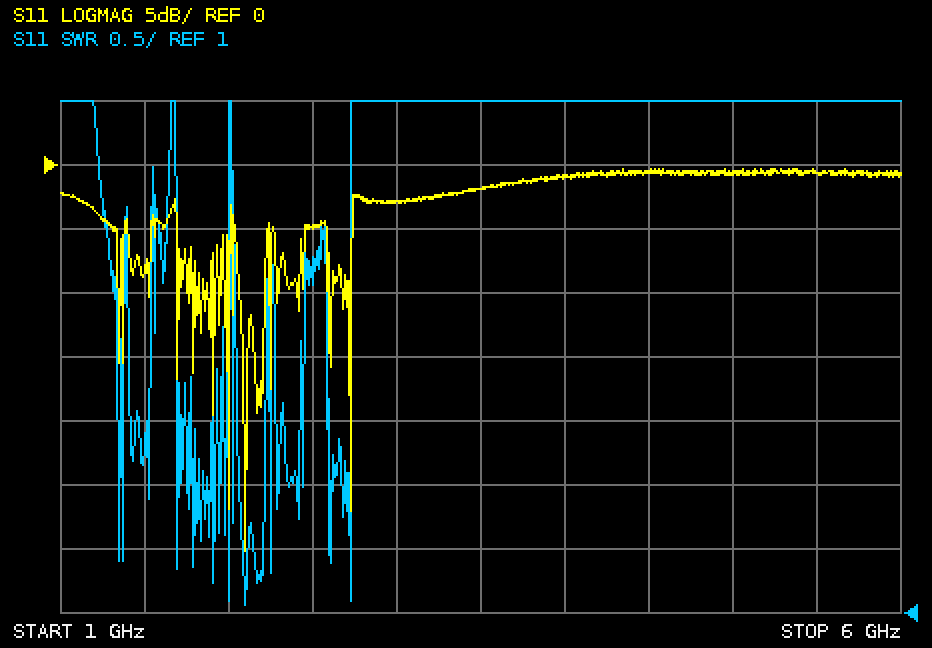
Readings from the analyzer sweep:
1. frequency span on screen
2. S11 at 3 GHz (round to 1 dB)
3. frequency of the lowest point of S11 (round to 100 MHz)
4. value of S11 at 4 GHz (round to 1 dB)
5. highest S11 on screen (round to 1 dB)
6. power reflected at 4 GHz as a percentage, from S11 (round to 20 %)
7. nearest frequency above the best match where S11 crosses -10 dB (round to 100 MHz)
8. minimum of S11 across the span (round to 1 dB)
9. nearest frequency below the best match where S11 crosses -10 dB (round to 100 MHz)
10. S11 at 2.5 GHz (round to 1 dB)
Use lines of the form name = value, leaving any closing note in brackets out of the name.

frequency span on screen = 5 GHz
S11 at 3 GHz = -3 dB
frequency of the lowest point of S11 = 2.1 GHz
value of S11 at 4 GHz = -1 dB
highest S11 on screen = 0 dB
power reflected at 4 GHz as a percentage, from S11 = 80 %
nearest frequency above the best match where S11 crosses -10 dB = 2.2 GHz
minimum of S11 across the span = -30 dB
nearest frequency below the best match where S11 crosses -10 dB = 2.1 GHz
S11 at 2.5 GHz = -5 dB
